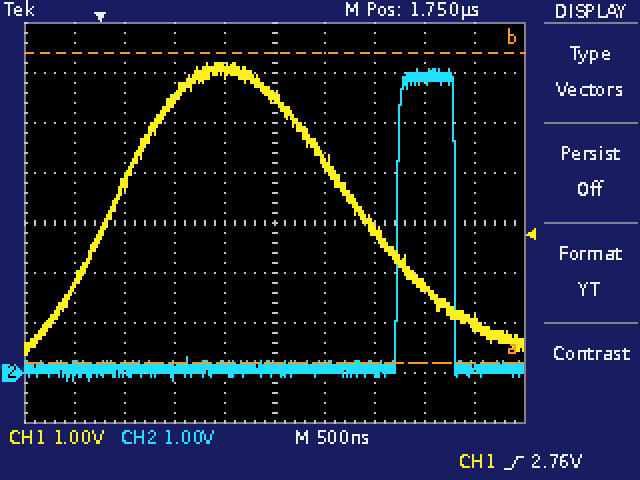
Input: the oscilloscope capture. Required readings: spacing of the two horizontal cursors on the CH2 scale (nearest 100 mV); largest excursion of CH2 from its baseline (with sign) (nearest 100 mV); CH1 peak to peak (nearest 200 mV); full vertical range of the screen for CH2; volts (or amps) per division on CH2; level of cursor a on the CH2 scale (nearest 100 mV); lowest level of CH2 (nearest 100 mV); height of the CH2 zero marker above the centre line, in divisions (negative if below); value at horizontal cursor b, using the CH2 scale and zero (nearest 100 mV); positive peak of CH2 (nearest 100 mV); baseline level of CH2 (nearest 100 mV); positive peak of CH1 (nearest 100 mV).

6.2 V
+6.0 V
5.8 V
8 V
1 V
200 mV
-200 mV
-3.0 div
6.4 V
6.1 V
100 mV
6.2 V
